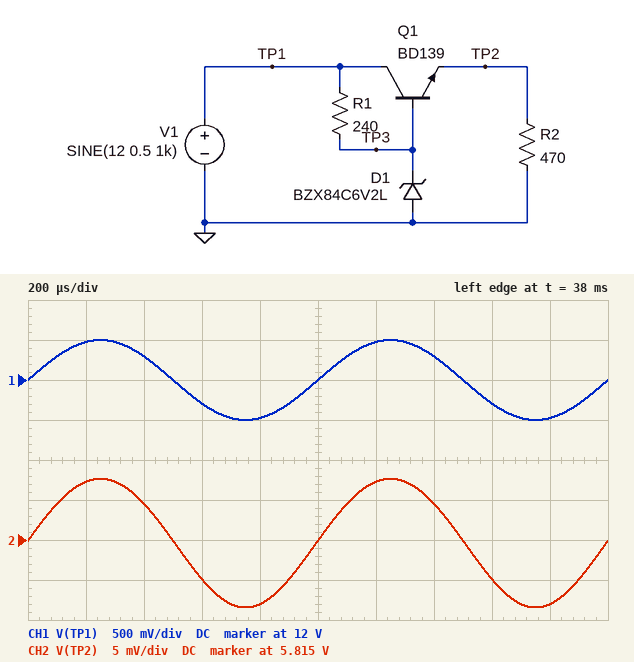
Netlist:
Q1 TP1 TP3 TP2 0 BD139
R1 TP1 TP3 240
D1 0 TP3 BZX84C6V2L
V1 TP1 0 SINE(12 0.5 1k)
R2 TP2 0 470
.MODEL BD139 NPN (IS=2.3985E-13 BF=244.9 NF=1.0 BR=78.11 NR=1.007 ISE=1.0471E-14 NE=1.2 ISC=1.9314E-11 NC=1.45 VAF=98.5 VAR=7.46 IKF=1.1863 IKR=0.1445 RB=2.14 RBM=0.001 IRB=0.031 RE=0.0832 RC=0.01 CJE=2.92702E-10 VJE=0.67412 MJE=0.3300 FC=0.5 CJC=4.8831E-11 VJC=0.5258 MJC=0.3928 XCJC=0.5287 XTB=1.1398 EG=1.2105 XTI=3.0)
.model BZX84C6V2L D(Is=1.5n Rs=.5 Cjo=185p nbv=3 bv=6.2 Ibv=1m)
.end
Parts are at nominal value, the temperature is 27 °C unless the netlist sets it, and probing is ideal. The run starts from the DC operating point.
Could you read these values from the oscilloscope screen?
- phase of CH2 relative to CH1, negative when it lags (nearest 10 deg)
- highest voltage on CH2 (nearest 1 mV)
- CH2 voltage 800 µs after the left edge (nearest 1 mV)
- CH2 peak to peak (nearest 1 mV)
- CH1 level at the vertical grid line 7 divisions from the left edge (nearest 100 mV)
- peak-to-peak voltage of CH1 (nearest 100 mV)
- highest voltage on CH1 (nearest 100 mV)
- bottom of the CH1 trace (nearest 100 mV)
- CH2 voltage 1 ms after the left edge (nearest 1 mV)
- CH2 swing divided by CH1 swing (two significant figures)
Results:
0 deg
5.823 V
5.807 V
16 mV
12.3 V
1.0 V
12.5 V
11.5 V
5.815 V
0.016
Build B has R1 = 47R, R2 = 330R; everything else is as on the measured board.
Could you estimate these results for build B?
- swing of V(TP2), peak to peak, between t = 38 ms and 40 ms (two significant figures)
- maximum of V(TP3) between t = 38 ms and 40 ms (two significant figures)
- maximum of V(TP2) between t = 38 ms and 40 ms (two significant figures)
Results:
25 mV
6.6 V
6.0 V
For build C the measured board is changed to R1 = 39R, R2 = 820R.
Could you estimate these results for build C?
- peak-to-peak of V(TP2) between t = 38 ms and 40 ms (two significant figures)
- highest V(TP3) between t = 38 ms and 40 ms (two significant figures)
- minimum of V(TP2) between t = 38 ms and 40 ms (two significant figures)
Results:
27 mV
6.7 V
6.0 V
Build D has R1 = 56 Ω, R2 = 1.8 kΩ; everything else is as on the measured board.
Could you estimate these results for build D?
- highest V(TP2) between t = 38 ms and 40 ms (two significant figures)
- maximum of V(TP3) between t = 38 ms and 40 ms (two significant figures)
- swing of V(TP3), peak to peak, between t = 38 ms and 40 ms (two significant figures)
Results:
6.0 V
6.6 V
23 mV
